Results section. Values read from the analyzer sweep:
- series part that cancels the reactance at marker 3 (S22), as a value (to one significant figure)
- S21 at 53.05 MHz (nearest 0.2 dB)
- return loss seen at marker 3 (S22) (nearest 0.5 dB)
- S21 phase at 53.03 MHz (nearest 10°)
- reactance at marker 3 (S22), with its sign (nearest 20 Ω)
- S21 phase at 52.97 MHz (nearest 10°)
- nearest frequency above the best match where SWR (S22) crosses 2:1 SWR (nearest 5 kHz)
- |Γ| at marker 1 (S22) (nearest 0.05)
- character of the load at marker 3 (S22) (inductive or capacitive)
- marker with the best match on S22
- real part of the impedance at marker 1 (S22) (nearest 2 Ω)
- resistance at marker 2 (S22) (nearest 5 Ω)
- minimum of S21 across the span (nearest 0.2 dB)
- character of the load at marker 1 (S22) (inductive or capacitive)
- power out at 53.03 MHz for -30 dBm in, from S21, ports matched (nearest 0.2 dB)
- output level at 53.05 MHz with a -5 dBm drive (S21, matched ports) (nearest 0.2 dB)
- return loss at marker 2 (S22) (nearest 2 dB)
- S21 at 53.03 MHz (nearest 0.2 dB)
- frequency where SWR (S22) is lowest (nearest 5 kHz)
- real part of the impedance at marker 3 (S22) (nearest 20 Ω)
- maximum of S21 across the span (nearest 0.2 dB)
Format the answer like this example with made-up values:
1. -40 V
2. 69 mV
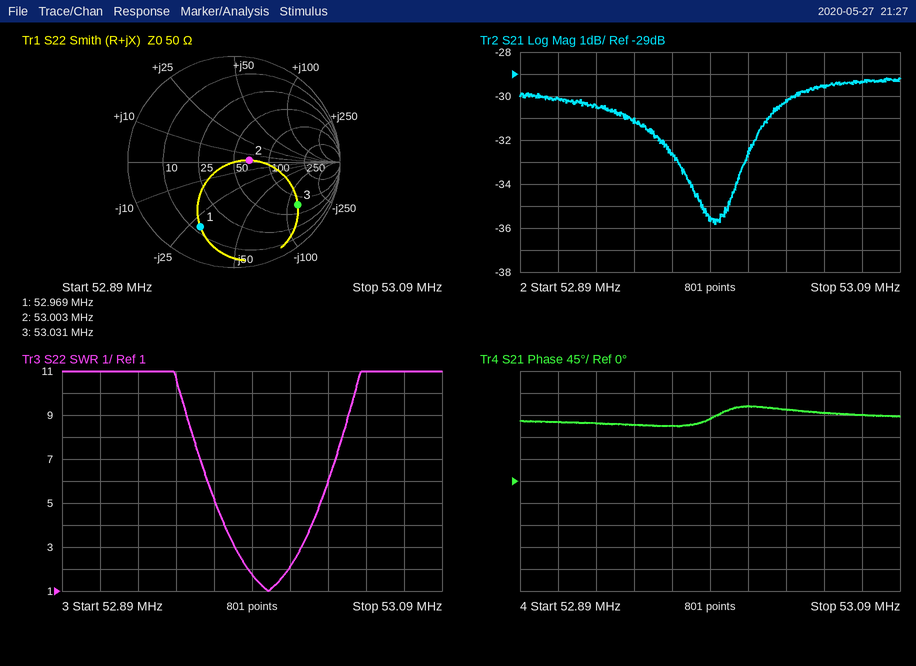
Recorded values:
1. 400 nH
2. -29.6 dB
3. 3.0 dB
4. 150°
5. -120 Ω
6. 110°
7. 53.010 MHz
8. 0.70
9. capacitive
10. marker 2
11. 12 Ω
12. 65 Ω
13. -35.8 dB
14. capacitive
15. -60.2 dBm
16. -34.6 dBm
17. 16 dB
18. -30.2 dB
19. 53.000 MHz
20. 80 Ω
21. -29.2 dB
